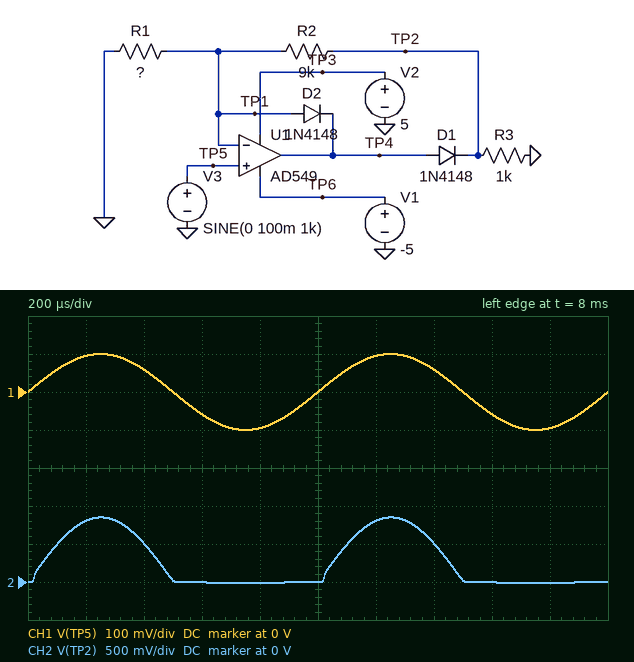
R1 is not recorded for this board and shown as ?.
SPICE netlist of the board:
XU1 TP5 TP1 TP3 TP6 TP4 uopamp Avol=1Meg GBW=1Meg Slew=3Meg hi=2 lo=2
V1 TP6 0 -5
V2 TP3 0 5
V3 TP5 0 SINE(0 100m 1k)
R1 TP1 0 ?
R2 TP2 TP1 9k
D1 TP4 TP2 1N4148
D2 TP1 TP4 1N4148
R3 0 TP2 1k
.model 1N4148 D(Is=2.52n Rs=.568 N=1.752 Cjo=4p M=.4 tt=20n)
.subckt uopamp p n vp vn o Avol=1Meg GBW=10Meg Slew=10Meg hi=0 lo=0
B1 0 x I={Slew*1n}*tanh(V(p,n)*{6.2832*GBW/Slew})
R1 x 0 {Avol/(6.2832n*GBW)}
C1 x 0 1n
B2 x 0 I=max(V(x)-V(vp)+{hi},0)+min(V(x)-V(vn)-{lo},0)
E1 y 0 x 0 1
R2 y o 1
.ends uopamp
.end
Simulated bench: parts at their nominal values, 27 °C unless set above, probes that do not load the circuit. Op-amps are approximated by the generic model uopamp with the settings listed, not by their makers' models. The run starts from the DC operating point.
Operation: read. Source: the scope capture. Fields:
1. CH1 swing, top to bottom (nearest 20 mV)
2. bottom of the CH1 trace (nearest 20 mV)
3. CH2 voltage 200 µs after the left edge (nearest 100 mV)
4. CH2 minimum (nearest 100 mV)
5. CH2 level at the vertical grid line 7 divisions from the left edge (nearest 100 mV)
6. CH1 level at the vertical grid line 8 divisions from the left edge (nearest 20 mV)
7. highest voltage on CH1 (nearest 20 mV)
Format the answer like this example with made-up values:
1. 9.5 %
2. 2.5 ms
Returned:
1. 200 mV
2. -100 mV
3. 800 mV
4. 0 V
5. 500 mV
6. -60 mV
7. 100 mV
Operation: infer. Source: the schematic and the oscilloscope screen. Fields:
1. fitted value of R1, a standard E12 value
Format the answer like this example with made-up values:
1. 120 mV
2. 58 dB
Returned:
1. 1.2 kΩ
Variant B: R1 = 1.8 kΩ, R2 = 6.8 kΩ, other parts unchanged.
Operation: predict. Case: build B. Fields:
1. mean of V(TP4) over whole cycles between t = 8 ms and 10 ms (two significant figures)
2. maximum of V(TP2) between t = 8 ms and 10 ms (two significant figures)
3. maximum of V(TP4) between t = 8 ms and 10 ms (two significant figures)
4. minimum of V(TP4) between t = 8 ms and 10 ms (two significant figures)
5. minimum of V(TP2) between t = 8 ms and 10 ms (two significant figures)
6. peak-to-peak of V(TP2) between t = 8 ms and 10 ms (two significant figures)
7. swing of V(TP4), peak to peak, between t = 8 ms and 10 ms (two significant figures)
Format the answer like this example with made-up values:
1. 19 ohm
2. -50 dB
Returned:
1. 170 mV
2. 480 mV
3. 1.0 V
4. -560 mV
5. -13 mV
6. 490 mV
7. 1.6 V
